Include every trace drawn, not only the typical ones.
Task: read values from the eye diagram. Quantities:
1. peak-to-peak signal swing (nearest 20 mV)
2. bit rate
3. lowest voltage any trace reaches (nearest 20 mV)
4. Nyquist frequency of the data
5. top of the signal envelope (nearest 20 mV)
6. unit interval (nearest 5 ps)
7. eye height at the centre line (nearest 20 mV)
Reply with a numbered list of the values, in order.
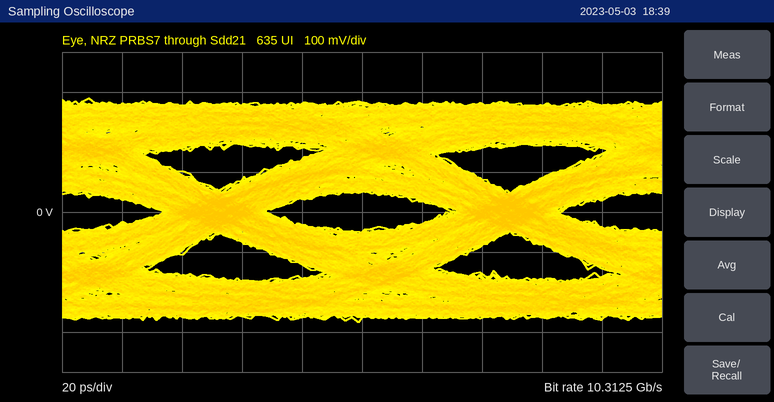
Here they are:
1. 560 mV
2. 10.3125 Gb/s
3. -280 mV
4. 5.15625 GHz
5. 280 mV
6. 95 ps
7. 100 mV
